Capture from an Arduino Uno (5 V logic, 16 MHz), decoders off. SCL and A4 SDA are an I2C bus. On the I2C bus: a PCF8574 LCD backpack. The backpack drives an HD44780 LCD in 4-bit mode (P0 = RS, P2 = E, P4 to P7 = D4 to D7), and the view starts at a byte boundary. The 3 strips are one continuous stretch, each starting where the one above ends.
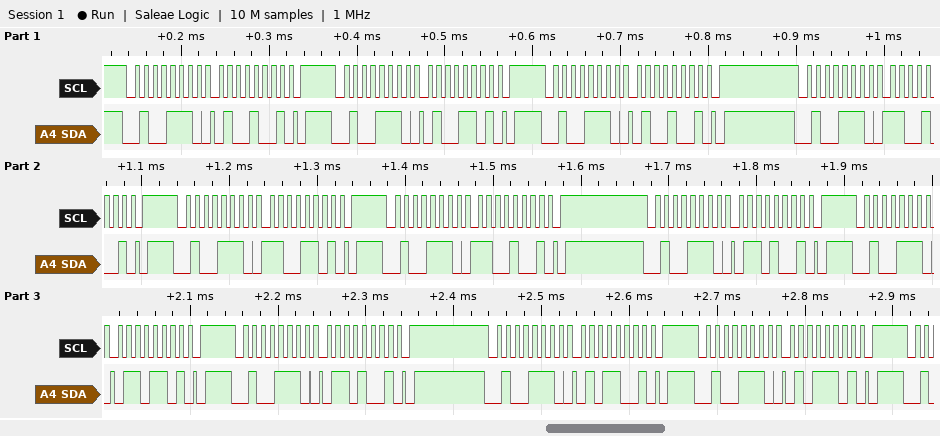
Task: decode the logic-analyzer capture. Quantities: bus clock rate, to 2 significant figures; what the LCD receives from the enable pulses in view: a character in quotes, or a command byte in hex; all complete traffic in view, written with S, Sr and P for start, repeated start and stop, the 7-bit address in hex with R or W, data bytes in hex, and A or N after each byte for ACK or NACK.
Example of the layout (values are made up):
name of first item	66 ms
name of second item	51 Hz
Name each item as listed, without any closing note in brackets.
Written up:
bus clock rate, to 2 significant figures	100 kHz
what the LCD receives from the enable pulses in view: a character in quotes, or a command byte in hex	'L'
all complete traffic in view, written with S, Sr and P for start, repeated start and stop, the 7-bit address in hex with R or W, data bytes in hex, and A or N after each byte for ACK or NACK	S 27W A 49 A P S 27W A 4D A P S 27W A 49 A P S 27W A C9 A P S 27W A CD A P S 27W A C9 A P S 27W A 69 A P S 27W A 6D A P S 27W A 69 A P S 27W A 59 A P S 27W A 5D A P
